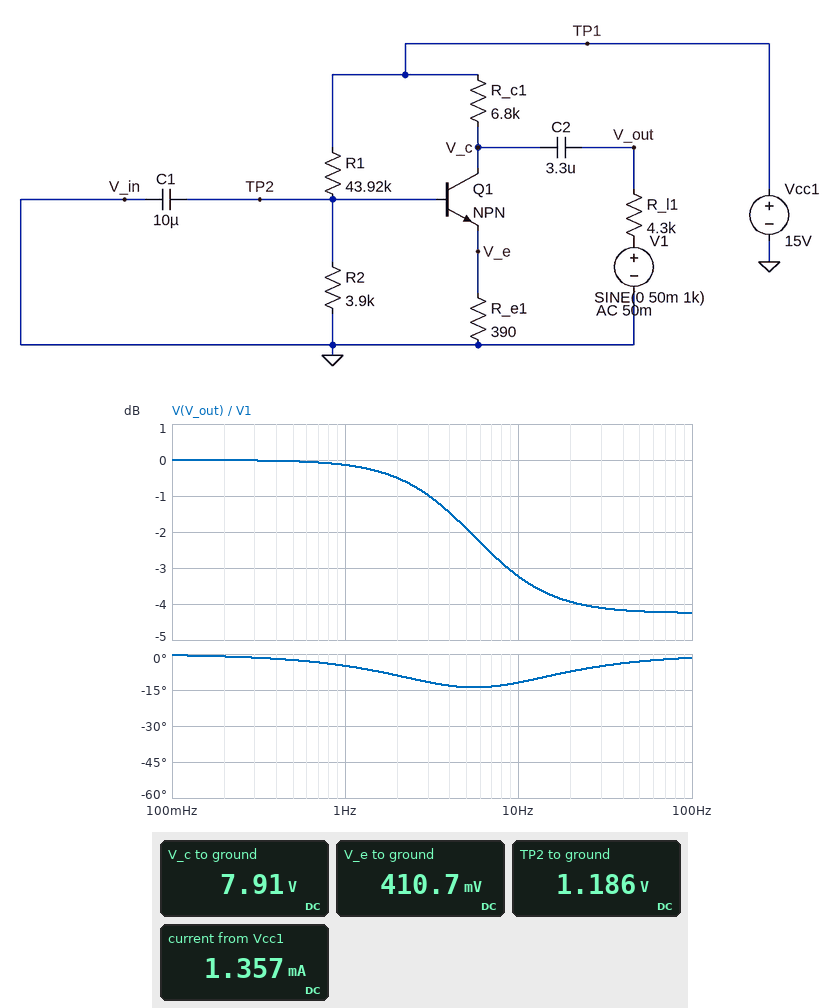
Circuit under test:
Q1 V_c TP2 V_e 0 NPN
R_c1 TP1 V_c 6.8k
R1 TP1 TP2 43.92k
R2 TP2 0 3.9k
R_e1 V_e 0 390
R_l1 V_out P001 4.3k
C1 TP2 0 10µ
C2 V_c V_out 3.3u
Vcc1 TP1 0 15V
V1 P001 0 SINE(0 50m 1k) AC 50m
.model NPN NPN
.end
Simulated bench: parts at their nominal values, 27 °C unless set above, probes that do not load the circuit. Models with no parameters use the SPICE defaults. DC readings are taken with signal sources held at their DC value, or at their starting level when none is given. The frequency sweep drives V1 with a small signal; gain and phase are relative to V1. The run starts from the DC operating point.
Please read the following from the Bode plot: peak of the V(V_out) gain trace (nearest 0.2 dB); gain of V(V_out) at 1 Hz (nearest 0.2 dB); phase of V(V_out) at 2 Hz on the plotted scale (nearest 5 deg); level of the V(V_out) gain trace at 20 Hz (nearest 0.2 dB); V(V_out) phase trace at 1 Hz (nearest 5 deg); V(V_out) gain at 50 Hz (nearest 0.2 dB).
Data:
0 dB
-0.2 dB
-10 deg
-4.0 dB
-5 deg
-4.2 dB
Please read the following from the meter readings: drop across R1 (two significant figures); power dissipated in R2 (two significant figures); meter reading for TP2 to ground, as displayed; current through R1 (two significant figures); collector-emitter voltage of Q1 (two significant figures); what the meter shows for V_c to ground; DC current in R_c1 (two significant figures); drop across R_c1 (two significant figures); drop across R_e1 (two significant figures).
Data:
14 V
360 µW
1.186 V
310 µA
7.5 V
7.91 V
1.0 mA
7.1 V
410 mV
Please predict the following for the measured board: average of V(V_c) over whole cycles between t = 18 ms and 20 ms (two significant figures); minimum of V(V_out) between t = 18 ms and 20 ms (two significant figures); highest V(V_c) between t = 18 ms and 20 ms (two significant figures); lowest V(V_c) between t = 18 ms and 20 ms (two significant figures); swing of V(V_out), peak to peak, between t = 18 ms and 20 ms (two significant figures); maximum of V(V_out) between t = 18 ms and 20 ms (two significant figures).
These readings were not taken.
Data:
7.9 V
-31 mV
7.9 V
7.9 V
61 mV
31 mV
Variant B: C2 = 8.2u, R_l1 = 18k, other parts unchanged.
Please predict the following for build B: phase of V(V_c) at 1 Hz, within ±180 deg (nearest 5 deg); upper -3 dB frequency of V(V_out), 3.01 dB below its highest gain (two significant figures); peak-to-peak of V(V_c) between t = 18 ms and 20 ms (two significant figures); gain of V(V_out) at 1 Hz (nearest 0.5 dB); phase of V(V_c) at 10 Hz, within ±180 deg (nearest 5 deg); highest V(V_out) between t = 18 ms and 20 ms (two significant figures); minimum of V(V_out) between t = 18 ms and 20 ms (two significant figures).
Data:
40 deg
850 mHz
27 mV
-3.5 dB
5 deg
14 mV
-14 mV
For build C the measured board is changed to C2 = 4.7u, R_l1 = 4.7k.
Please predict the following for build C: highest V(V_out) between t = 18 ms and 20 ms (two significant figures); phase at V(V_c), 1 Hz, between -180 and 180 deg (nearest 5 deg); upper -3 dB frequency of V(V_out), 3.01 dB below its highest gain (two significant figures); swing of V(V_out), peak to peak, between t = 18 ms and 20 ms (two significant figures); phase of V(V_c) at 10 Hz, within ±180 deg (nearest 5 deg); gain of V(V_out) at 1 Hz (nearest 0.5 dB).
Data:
30 mV
70 deg
5.4 Hz
59 mV
15 deg
-0.5 dB
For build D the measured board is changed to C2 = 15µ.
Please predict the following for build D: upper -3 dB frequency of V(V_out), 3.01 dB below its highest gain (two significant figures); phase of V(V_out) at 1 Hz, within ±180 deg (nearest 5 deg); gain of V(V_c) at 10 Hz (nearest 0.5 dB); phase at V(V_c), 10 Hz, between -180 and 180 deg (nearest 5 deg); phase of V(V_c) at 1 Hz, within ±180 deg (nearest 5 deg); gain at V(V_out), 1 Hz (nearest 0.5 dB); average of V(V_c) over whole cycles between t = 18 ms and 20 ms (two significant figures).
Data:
1.9 Hz
-15 deg
-4.5 dB
5 deg
45 deg
-1.5 dB
7.9 V
